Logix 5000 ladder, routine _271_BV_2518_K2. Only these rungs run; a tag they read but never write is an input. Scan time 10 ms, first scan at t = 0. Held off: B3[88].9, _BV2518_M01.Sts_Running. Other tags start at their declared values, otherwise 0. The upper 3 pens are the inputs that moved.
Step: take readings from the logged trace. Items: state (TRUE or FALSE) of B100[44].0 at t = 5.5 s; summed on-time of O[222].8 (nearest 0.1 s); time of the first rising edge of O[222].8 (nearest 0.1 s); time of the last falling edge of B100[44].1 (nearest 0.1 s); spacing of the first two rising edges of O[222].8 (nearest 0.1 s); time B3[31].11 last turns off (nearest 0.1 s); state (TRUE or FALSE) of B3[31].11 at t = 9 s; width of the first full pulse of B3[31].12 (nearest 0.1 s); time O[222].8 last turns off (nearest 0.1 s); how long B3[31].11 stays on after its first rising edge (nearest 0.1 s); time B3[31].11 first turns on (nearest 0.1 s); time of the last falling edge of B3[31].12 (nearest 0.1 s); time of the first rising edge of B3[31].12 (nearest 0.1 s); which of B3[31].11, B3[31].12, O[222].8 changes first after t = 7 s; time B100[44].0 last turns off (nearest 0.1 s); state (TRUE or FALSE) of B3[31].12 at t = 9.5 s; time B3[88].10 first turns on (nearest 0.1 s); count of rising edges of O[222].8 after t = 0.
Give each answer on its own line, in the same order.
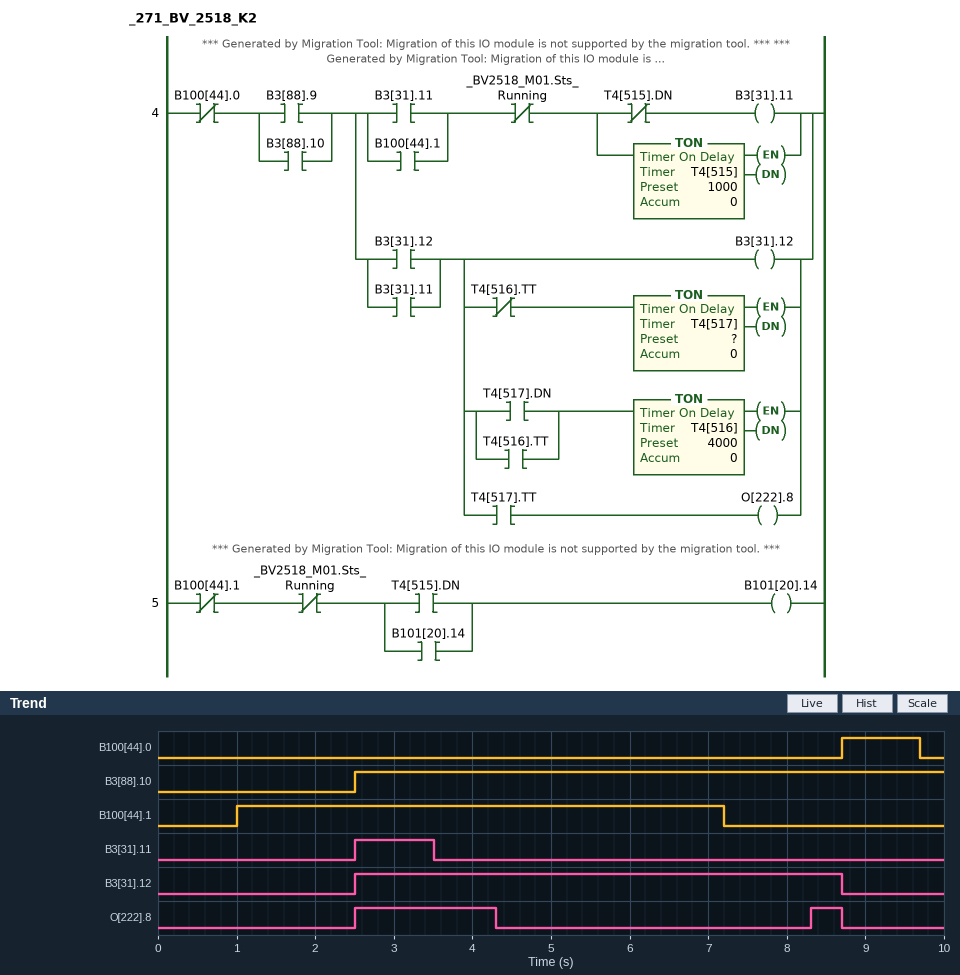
FALSE
2.2 s
2.5 s
7.2 s
5.8 s
3.5 s
FALSE
6.2 s
8.7 s
1.0 s
2.5 s
8.7 s
2.5 s
O[222].8
9.7 s
FALSE
2.5 s
2
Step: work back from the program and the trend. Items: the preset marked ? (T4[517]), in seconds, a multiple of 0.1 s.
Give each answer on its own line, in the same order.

1.8 s
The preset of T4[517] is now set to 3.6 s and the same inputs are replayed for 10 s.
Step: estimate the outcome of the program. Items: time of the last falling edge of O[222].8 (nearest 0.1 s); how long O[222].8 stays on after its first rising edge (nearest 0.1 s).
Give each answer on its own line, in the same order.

6.1 s
3.6 s
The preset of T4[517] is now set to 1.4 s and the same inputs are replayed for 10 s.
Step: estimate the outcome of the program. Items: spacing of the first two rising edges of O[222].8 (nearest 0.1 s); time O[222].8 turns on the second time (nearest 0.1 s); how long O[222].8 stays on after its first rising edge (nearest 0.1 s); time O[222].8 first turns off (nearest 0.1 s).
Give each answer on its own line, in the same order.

5.4 s
7.9 s
1.4 s
3.9 s
